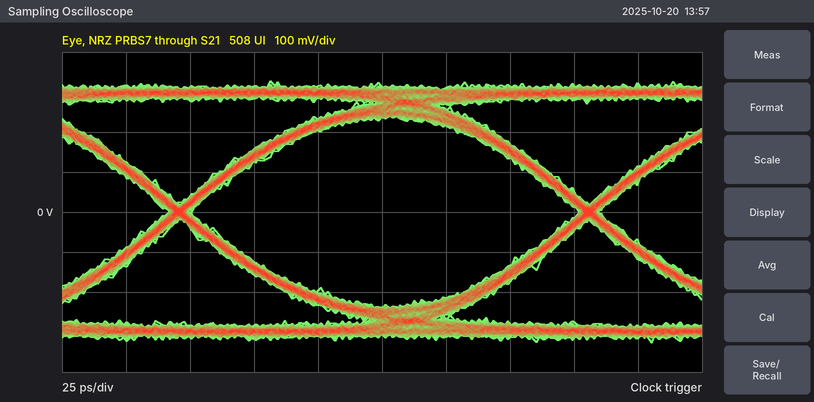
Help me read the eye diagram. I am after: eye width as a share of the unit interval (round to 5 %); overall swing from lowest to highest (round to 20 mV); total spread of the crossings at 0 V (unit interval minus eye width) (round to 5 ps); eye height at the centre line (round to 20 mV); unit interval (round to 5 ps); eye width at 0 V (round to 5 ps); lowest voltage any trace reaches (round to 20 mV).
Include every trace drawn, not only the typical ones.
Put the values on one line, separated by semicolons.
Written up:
95 %; 660 mV; 10 ps; 480 mV; 160 ps; 150 ps; -320 mV
